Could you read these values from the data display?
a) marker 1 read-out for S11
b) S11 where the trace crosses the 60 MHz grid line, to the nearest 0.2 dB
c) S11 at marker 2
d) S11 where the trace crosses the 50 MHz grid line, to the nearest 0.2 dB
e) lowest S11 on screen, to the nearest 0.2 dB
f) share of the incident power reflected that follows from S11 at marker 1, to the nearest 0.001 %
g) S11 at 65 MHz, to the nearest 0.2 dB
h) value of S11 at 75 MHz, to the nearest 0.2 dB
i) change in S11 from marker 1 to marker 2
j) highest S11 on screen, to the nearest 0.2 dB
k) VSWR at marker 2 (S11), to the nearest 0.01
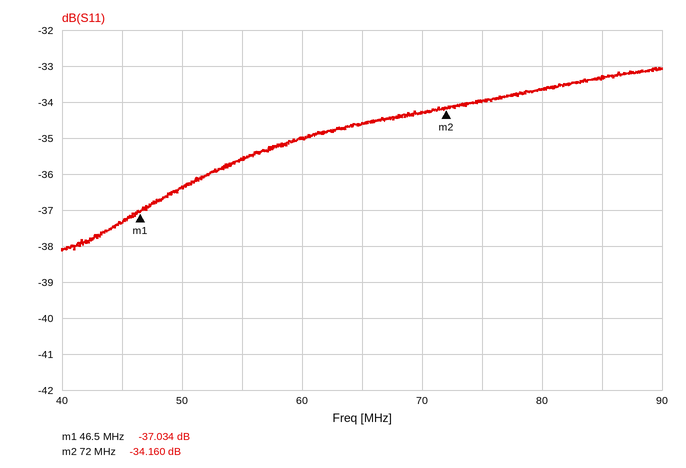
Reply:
-37.034 dB
-35.0 dB
-34.160 dB
-36.4 dB
-38.2 dB
0.020 %
-34.6 dB
-34.0 dB
2.874 dB
-33.0 dB
1.04
